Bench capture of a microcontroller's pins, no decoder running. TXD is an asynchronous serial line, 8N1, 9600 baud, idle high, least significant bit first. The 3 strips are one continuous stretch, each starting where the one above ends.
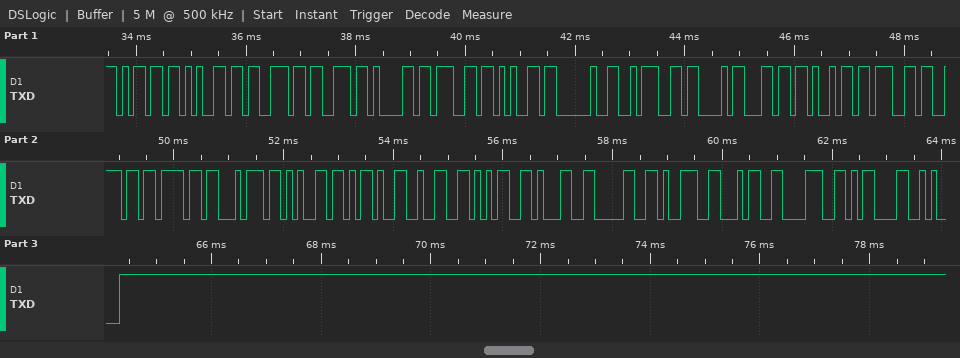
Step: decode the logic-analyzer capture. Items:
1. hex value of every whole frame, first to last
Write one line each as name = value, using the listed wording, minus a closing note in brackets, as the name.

hex value of every whole frame, first to last = 6D 65 73 73 61 67 65 20 3A 43 6C 69 67 6E 6F 74 65 2D 32 35 31 30 39 34 38 0D 0A
